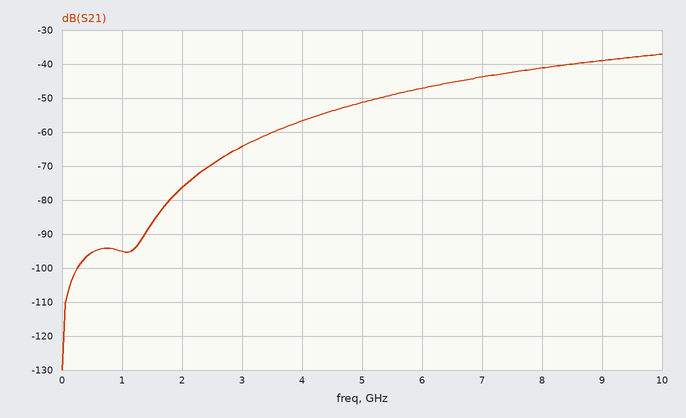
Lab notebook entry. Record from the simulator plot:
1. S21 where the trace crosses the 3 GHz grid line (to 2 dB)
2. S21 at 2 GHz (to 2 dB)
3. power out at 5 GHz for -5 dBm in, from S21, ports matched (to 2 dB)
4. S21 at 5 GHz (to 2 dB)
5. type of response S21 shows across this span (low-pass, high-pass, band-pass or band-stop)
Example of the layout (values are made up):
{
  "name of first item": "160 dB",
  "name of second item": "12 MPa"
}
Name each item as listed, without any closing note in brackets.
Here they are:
{
  "S21 where the trace crosses the 3 GHz grid line": "-64 dB",
  "S21 at 2 GHz": "-76 dB",
  "power out at 5 GHz for -5 dBm in, from S21, ports matched": "-56 dBm",
  "S21 at 5 GHz": "-52 dB",
  "type of response S21 shows across this span": "high-pass"
}
